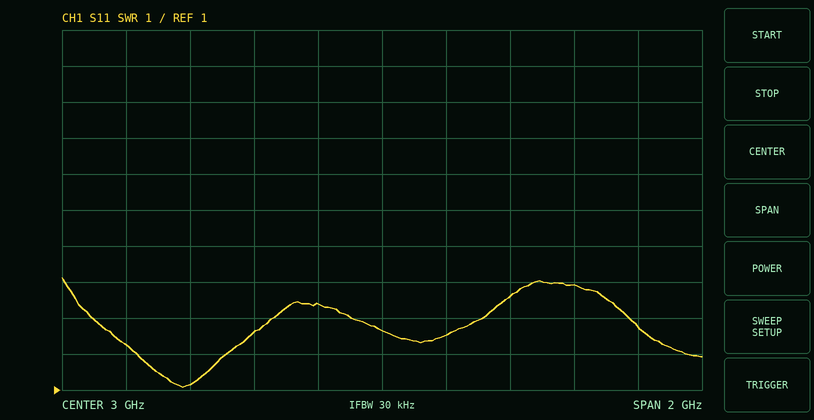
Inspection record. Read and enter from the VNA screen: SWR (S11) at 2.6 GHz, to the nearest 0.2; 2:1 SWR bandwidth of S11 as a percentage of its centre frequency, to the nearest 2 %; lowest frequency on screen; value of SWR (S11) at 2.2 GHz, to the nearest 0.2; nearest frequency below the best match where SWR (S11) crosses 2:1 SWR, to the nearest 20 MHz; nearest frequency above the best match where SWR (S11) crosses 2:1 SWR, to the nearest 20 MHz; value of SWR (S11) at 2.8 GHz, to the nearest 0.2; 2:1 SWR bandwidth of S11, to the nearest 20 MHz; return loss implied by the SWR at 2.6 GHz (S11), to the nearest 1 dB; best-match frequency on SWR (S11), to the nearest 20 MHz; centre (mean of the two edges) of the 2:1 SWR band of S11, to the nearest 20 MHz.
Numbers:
2.6
12 %
2 GHz
2.2
2.24 GHz
2.52 GHz
3.4
280 MHz
7 dB
2.38 GHz
2.38 GHz
